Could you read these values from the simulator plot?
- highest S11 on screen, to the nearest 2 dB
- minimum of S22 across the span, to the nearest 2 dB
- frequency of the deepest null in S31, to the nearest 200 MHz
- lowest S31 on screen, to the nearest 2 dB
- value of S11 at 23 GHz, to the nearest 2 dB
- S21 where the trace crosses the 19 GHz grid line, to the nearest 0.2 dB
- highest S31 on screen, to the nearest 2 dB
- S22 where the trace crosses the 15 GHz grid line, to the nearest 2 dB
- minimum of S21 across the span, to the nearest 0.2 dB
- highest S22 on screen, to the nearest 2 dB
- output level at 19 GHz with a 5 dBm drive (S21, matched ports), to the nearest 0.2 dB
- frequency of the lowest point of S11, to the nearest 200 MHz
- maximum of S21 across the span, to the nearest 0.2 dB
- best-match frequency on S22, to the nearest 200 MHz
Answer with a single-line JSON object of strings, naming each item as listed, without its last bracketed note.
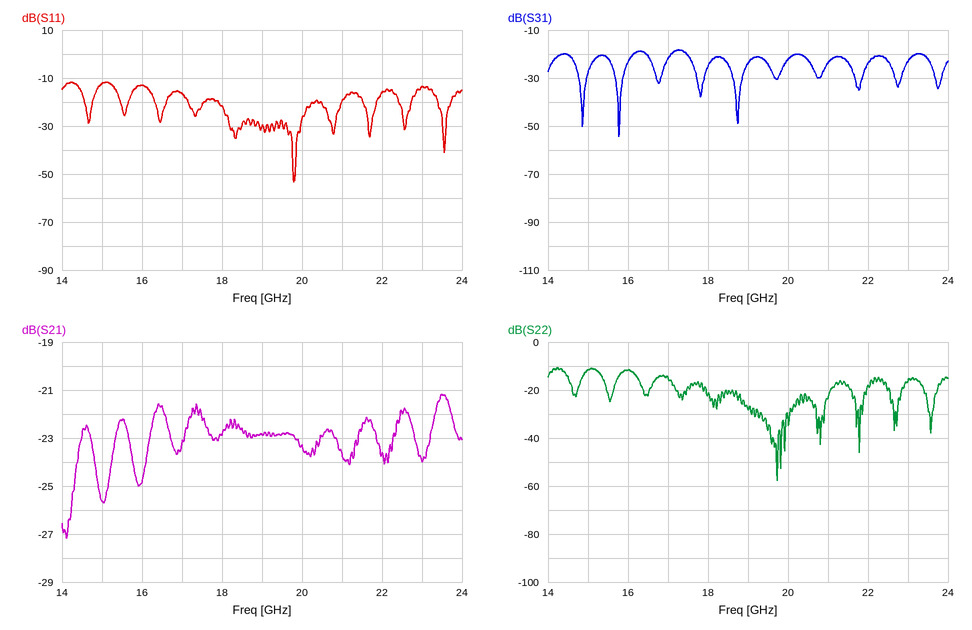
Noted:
{"highest S11 on screen, to the nearest 2 dB": "-12 dB", "minimum of S22 across the span, to the nearest 2 dB": "-58 dB", "frequency of the deepest null in S31, to the nearest 200 MHz": "15.8 GHz", "lowest S31 on screen, to the nearest 2 dB": "-54 dB", "value of S11 at 23 GHz, to the nearest 2 dB": "-14 dB", "S21 where the trace crosses the 19 GHz grid line, to the nearest 0.2 dB": "-22.8 dB", "highest S31 on screen, to the nearest 2 dB": "-18 dB", "S22 where the trace crosses the 15 GHz grid line, to the nearest 2 dB": "-12 dB", "minimum of S21 across the span, to the nearest 0.2 dB": "-27.2 dB", "highest S22 on screen, to the nearest 2 dB": "-10 dB", "output level at 19 GHz with a 5 dBm drive (S21, matched ports), to the nearest 0.2 dB": "-17.8 dBm", "frequency of the lowest point of S11, to the nearest 200 MHz": "19.8 GHz", "maximum of S21 across the span, to the nearest 0.2 dB": "-21.2 dB", "best-match frequency on S22, to the nearest 200 MHz": "19.8 GHz"}
